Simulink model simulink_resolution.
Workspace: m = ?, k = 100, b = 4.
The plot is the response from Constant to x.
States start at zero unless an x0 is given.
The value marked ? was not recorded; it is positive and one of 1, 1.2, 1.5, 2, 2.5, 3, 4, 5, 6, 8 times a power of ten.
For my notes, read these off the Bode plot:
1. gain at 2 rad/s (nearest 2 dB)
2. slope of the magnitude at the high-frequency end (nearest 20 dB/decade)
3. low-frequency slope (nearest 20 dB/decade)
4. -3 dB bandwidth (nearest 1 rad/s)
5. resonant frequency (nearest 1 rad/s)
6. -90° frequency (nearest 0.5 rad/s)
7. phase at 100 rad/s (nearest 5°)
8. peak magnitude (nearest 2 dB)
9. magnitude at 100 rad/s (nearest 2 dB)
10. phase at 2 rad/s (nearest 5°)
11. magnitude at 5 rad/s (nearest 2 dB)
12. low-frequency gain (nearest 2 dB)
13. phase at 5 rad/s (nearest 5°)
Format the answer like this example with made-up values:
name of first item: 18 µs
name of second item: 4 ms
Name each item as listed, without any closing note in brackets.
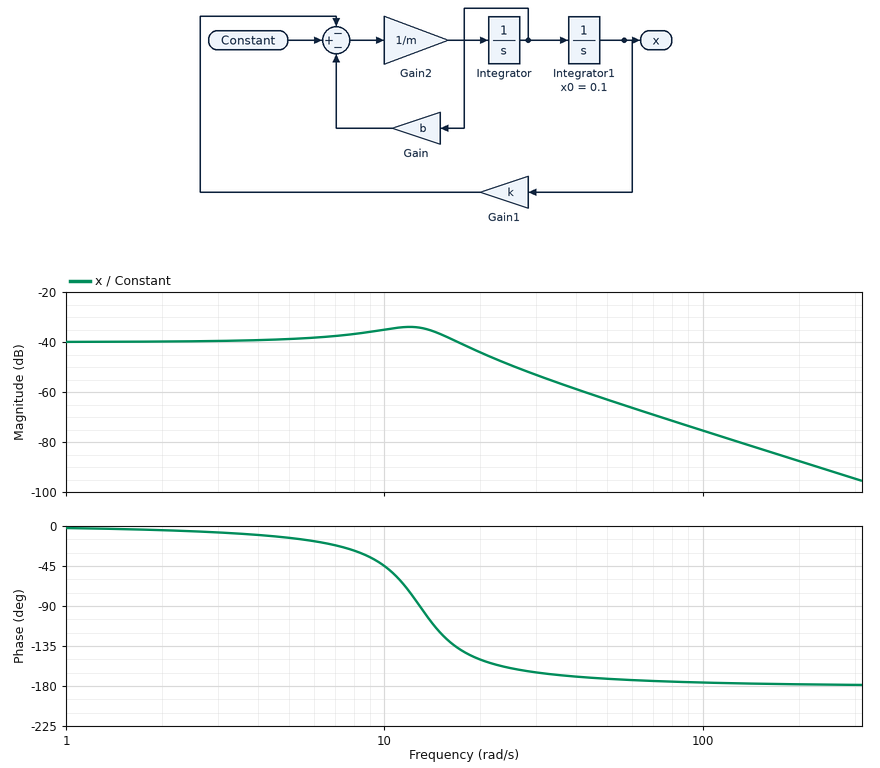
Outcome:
gain at 2 rad/s: -40 dB
slope of the magnitude at the high-frequency end: -40 dB/decade
low-frequency slope: 0 dB/decade
-3 dB bandwidth: 19 rad/s
resonant frequency: 12 rad/s
-90° frequency: 13.0 rad/s
phase at 100 rad/s: -175°
peak magnitude: -34 dB
magnitude at 100 rad/s: -76 dB
phase at 2 rad/s: -5°
magnitude at 5 rad/s: -38 dB
low-frequency gain: -40 dB
phase at 5 rad/s: -15°
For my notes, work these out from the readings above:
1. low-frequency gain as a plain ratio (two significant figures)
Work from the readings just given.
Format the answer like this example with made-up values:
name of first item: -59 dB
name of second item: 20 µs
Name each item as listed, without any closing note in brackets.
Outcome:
low-frequency gain as a plain ratio: 0.010
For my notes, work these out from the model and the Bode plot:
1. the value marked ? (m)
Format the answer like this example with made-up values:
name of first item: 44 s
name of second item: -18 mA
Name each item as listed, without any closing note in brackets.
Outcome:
the value marked ?: 0.6
